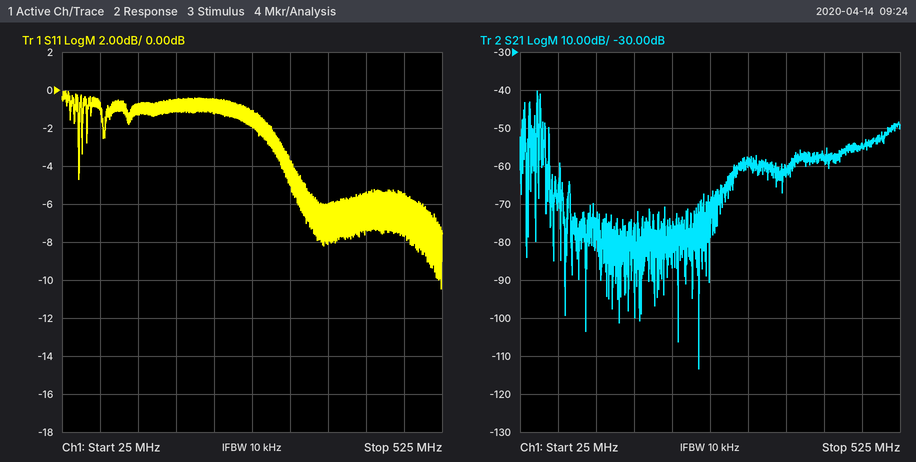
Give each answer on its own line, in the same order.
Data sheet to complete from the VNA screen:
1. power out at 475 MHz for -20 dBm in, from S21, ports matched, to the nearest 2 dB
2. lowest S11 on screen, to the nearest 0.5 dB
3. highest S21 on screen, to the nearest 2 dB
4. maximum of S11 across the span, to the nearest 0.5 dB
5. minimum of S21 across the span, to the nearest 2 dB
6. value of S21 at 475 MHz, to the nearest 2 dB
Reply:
-74 dBm
-10.5 dB
-40 dB
0.0 dB
-114 dB
-54 dB
